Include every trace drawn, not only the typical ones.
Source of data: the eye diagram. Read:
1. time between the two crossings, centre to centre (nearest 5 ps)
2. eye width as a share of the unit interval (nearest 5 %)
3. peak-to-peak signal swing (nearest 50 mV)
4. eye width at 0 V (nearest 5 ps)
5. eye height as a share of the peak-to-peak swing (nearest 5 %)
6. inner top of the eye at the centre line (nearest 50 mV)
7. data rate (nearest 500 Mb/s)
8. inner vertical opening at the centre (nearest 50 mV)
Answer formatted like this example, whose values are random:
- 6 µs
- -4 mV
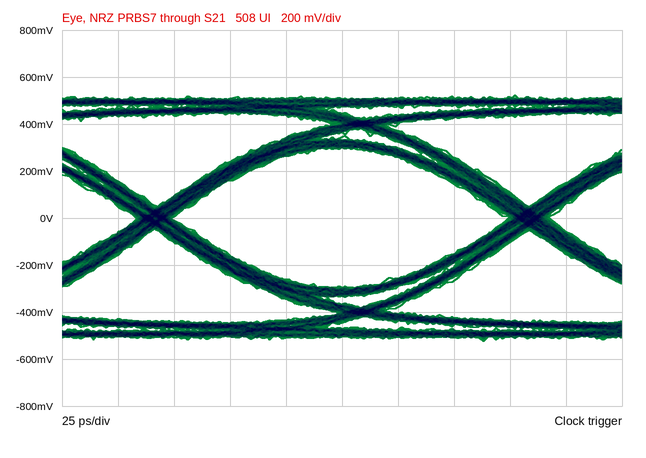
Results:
- 165 ps
- 90 %
- 1.05 V
- 150 ps
- 55 %
- 300 mV
- 6.0 Gb/s
- 600 mV
